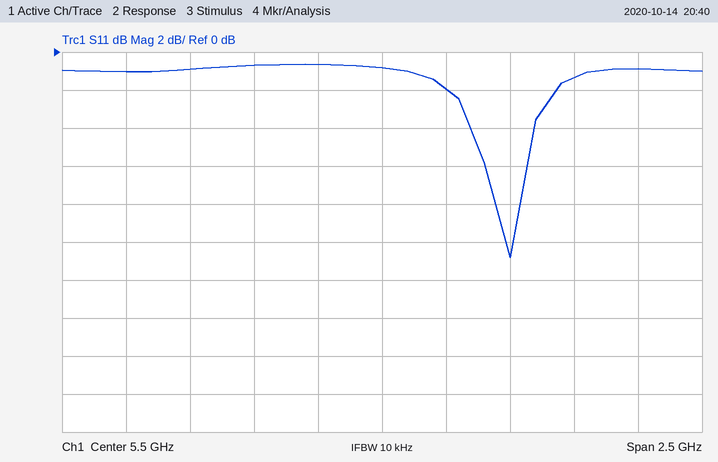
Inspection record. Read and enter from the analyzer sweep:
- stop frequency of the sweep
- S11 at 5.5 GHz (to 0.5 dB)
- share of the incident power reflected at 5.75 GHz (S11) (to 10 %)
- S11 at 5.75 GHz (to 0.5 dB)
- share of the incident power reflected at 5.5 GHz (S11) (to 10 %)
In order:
6.75 GHz
-1.0 dB
60 %
-2.0 dB
80 %
